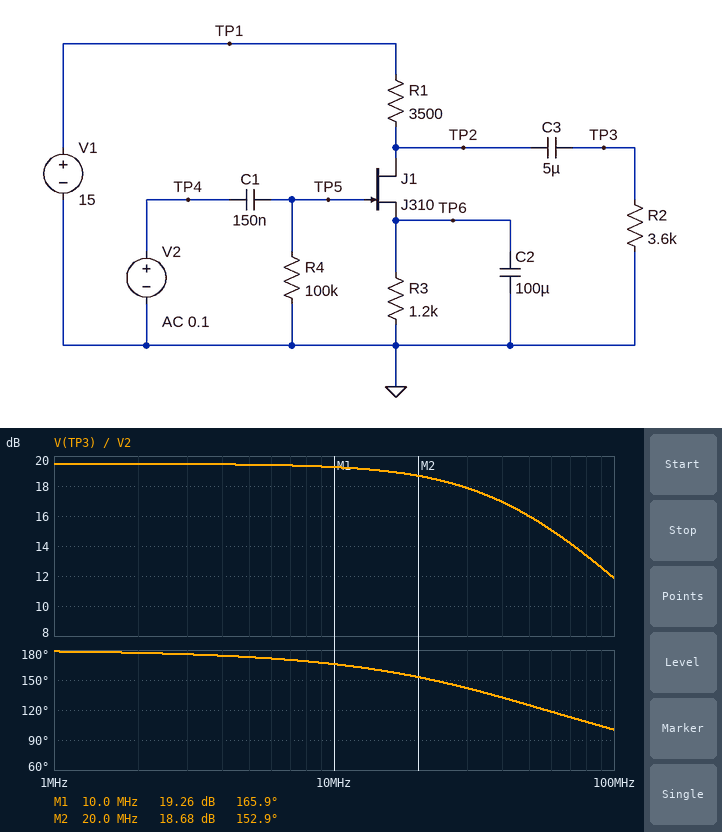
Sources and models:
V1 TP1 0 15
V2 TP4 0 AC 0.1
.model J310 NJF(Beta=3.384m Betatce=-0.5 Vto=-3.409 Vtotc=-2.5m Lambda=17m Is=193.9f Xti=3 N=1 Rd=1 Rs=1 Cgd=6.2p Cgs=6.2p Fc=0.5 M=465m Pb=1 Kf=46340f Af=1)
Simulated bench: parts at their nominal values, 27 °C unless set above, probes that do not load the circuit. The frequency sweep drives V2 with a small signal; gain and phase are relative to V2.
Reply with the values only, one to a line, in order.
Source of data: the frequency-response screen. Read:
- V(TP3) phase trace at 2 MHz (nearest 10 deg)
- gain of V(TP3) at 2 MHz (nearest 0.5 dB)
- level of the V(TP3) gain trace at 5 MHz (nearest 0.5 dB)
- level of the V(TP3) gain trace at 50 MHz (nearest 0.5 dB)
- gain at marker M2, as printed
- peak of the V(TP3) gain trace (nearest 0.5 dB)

180 deg
19.5 dB
19.5 dB
16.0 dB
18.68 dB
19.5 dB
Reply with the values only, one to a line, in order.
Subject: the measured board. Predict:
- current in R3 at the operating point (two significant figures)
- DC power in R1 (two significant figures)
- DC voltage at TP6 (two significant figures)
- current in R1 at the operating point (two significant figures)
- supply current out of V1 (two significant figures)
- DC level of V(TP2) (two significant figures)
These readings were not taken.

2.2 mA
17 mW
2.6 V
2.2 mA
2.2 mA
7.3 V
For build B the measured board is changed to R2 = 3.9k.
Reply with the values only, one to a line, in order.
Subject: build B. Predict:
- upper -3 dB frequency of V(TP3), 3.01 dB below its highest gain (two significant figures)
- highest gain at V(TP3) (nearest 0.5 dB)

43 MHz
20.0 dB
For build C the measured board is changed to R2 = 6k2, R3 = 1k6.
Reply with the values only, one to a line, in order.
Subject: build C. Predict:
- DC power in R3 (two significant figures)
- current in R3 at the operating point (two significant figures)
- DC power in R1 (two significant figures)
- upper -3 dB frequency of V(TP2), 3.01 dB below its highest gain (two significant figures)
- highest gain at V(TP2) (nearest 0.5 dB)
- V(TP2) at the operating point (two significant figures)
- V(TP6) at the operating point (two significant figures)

4.7 mW
1.7 mA
10 mW
39 MHz
20.5 dB
9.0 V
2.7 V
